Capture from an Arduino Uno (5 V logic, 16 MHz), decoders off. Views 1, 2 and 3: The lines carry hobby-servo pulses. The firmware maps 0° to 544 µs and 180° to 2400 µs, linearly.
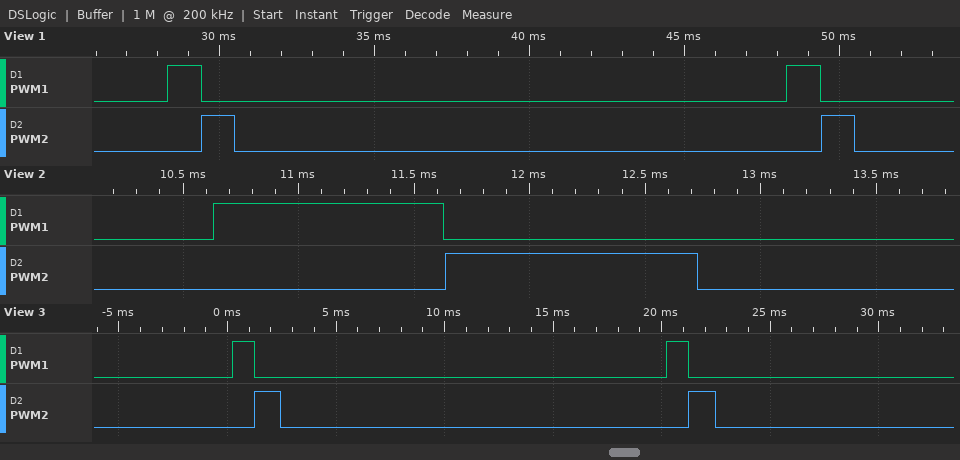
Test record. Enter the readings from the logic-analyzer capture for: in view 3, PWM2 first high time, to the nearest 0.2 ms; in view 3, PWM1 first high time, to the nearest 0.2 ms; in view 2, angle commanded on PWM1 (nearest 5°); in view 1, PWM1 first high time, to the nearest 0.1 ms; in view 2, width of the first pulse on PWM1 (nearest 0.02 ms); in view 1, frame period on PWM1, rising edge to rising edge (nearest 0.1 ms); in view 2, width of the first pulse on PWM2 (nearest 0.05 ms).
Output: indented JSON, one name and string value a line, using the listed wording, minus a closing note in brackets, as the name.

{
  "in view 3, PWM2 first high time, to the nearest 0.2 ms": "1.2 ms",
  "in view 3, PWM1 first high time, to the nearest 0.2 ms": "1.0 ms",
  "in view 2, angle commanded on PWM1": "45°",
  "in view 1, PWM1 first high time, to the nearest 0.1 ms": "1.1 ms",
  "in view 2, width of the first pulse on PWM1": "1.00 ms",
  "in view 1, frame period on PWM1, rising edge to rising edge": "20.0 ms",
  "in view 2, width of the first pulse on PWM2": "1.10 ms"
}
